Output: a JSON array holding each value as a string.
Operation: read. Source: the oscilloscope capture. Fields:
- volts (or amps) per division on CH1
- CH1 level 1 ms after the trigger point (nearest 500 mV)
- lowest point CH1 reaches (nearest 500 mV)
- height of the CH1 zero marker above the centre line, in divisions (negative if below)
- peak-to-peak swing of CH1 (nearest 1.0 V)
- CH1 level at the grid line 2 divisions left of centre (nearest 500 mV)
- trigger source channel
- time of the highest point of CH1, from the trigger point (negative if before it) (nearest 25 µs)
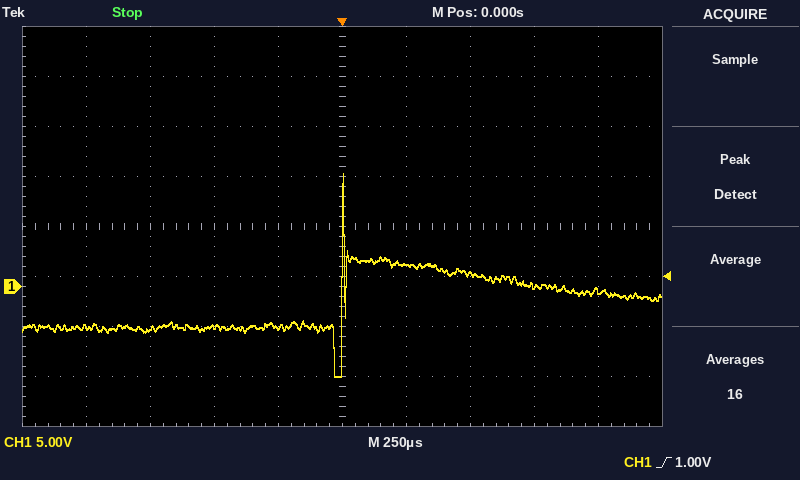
["5 V", "-500 mV", "-9.0 V", "-1.2 div", "20.0 V", "-4.0 V", "CH1", "0 µs"]
